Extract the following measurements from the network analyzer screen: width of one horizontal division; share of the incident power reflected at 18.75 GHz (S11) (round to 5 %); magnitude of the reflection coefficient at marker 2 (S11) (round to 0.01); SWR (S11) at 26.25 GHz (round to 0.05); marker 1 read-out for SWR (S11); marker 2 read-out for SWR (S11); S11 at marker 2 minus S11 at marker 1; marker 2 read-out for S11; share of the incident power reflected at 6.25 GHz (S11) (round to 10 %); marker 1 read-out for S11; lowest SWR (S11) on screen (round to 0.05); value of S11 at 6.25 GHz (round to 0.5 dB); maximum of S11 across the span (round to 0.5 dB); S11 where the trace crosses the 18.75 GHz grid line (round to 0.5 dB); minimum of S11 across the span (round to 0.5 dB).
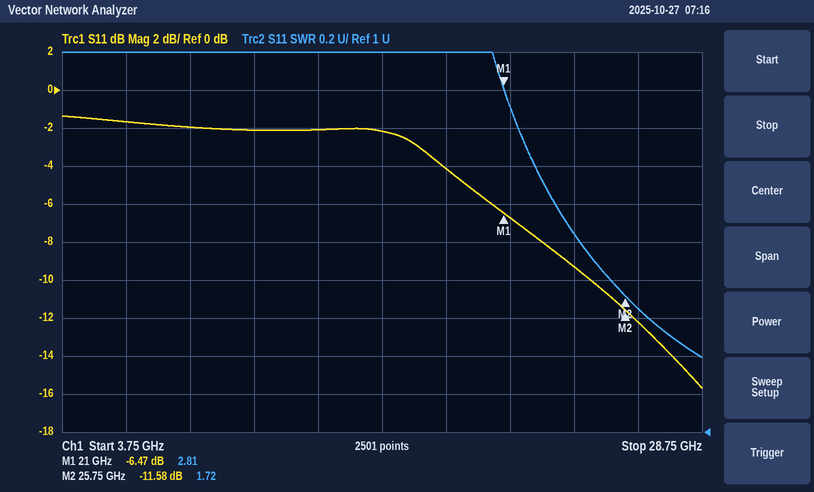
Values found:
2.5 GHz
40 %
0.26
1.65
2.81
1.72
-5.11 dB
-11.58 dB
70 %
-6.47 dB
1.40
-1.5 dB
-1.5 dB
-4.0 dB
-15.5 dB
